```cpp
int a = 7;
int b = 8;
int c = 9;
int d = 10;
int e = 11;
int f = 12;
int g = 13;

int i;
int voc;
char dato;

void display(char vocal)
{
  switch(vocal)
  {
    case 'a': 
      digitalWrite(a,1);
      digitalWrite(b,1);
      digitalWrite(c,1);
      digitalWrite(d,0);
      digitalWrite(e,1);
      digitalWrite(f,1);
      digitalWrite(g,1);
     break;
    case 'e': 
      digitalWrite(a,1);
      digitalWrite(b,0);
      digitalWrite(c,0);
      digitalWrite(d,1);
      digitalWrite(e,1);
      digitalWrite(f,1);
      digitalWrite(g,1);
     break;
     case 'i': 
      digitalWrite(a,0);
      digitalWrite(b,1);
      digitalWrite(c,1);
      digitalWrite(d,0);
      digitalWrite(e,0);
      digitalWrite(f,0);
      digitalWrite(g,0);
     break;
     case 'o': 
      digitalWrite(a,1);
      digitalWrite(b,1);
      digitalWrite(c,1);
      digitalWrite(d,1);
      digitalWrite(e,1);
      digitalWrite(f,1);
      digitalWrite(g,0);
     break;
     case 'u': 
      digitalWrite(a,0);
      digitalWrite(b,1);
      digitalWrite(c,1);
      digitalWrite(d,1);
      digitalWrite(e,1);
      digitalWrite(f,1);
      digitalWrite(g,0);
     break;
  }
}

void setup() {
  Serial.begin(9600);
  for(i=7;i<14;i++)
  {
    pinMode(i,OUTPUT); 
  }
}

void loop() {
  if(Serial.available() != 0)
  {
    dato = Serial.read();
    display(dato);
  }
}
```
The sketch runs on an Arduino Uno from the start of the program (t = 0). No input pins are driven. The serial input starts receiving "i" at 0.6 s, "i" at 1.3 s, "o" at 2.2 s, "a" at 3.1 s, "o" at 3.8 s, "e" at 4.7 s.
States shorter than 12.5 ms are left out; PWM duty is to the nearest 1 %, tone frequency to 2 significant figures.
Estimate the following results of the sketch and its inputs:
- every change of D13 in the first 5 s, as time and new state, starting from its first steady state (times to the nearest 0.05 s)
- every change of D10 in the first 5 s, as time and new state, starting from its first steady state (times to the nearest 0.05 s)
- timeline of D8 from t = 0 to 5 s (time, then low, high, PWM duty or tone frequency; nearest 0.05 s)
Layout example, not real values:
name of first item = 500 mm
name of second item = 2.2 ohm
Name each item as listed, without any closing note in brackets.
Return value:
every change of D13 in the first 5 s, as time and new state, starting from its first steady state = 0 s low; 3.1 s high; 3.8 s low; 4.7 s high
every change of D10 in the first 5 s, as time and new state, starting from its first steady state = 0 s low; 2.2 s high; 3.1 s low; 3.8 s high
timeline of D8 from t = 0 to 5 s = 0 s low; 0.6 s high; 4.7 s low
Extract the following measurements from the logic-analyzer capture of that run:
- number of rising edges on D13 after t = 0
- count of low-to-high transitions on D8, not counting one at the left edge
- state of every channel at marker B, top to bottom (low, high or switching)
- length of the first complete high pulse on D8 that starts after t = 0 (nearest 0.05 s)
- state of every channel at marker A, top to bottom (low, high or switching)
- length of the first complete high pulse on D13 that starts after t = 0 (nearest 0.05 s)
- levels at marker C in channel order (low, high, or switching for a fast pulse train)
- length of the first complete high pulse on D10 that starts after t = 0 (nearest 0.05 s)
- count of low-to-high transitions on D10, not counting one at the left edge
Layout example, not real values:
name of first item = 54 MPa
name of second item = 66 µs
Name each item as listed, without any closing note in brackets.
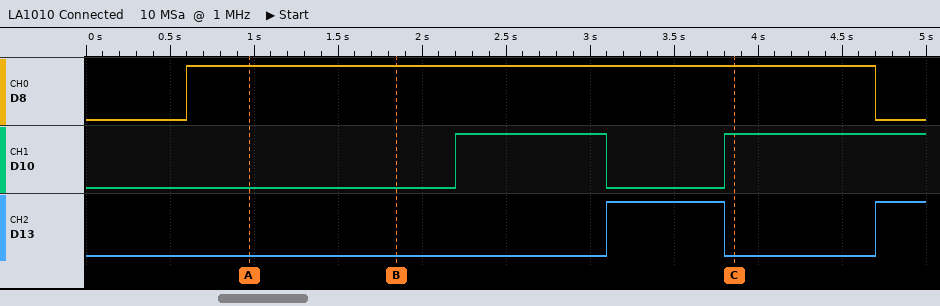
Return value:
number of rising edges on D13 after t = 0 = 2
count of low-to-high transitions on D8, not counting one at the left edge = 1
state of every channel at marker B, top to bottom = D8 high, D10 low, D13 low
length of the first complete high pulse on D8 that starts after t = 0 = 4.10 s
state of every channel at marker A, top to bottom = D8 high, D10 low, D13 low
length of the first complete high pulse on D13 that starts after t = 0 = 0.70 s
levels at marker C in channel order = D8 high, D10 high, D13 low
length of the first complete high pulse on D10 that starts after t = 0 = 0.90 s
count of low-to-high transitions on D10, not counting one at the left edge = 2
